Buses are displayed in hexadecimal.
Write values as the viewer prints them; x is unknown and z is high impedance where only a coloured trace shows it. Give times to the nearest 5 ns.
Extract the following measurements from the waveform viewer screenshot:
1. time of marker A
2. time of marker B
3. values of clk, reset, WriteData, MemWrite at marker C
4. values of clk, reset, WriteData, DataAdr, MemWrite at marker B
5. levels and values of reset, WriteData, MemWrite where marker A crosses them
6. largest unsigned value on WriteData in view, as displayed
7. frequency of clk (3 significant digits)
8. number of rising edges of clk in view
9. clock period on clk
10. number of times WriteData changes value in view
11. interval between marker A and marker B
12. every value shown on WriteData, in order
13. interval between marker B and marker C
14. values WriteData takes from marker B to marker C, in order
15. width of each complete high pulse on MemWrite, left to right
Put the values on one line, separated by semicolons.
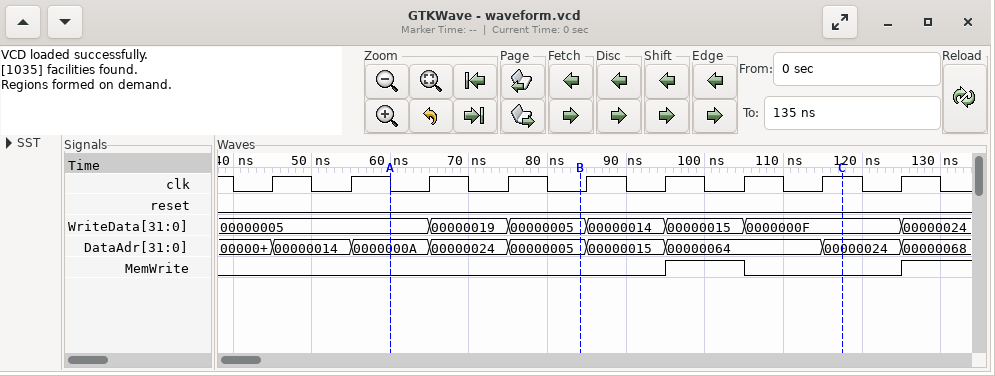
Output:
60 ns; 85 ns; clk=1, reset=0, WriteData=0000000F, MemWrite=0; clk=0, reset=0, WriteData=00000005, DataAdr=00000005, MemWrite=0; reset=0, WriteData=00000005, MemWrite=0; 00000024; 100 MHz; 9; 10 ns; 6; 25 ns; 00000005, 00000019, 00000005, 00000014, 00000015, 0000000F, 00000024; 35 ns; 00000005, 00000014, 00000015, 0000000F; 10 ns
